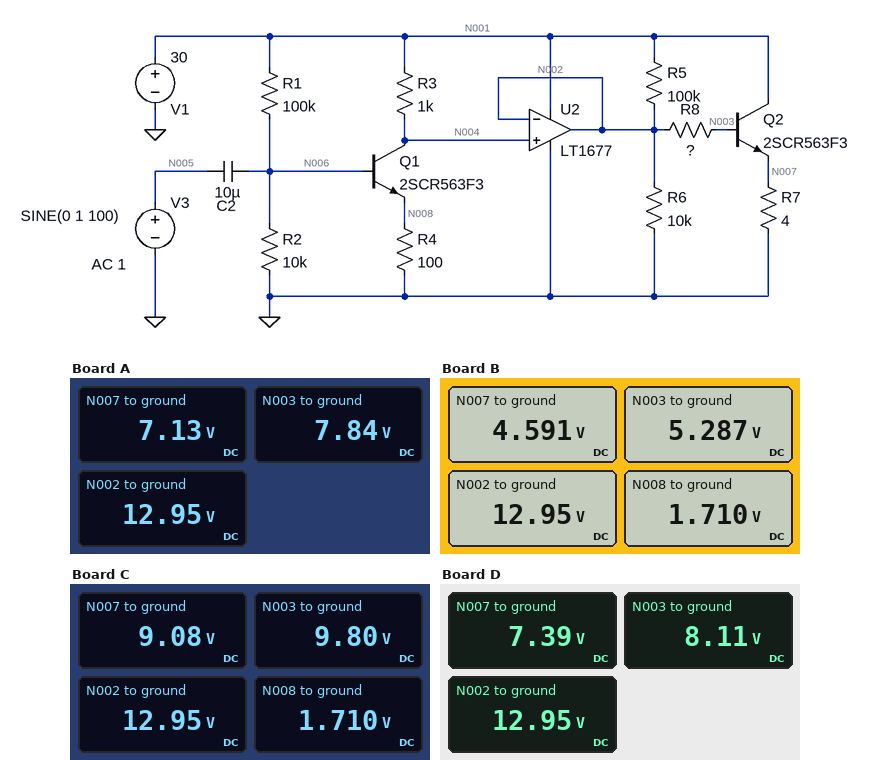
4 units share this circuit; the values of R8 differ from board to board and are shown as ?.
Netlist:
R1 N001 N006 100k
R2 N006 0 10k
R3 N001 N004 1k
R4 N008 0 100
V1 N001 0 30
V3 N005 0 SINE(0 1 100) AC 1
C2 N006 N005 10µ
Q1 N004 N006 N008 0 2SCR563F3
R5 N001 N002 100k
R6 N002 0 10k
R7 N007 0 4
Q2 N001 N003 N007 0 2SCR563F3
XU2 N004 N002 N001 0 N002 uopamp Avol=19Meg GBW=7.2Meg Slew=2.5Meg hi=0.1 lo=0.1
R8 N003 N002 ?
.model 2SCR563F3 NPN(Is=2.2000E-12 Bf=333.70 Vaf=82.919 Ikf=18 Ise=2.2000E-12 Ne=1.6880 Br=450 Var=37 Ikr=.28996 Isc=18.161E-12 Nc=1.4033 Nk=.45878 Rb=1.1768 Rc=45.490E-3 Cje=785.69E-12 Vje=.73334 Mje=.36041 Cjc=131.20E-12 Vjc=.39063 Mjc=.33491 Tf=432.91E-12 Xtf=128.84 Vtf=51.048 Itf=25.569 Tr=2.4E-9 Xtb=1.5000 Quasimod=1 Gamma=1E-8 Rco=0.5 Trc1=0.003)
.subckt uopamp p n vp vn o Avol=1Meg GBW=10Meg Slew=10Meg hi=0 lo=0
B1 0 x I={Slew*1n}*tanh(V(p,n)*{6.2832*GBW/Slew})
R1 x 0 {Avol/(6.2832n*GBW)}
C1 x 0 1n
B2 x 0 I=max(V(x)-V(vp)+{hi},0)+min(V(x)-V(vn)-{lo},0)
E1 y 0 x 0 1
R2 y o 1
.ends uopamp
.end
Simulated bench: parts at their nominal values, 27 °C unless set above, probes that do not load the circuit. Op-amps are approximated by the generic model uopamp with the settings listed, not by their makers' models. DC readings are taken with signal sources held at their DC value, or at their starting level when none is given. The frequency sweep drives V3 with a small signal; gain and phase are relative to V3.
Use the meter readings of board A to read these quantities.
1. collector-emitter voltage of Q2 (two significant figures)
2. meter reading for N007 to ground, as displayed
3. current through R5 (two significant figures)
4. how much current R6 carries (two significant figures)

23 V
7.13 V
170 µA
1.3 mA
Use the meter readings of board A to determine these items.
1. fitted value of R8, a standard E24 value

1.1 kΩ
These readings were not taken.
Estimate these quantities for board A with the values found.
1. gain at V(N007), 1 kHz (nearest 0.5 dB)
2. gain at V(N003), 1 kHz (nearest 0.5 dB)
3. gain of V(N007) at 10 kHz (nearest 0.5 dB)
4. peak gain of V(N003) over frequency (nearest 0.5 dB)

14.5 dB
14.5 dB
14.5 dB
14.5 dB
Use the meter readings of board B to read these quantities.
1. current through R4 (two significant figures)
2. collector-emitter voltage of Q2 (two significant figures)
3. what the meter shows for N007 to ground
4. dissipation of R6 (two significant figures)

17 mA
25 V
4.591 V
17 mW
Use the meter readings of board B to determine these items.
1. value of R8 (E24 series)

2.7 kΩ
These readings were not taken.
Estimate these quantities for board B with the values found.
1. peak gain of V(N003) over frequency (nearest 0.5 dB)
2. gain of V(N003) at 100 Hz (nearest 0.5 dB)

11.0 dB
11.0 dB
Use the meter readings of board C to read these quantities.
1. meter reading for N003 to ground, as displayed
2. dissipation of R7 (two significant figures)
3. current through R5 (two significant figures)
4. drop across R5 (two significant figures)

9.80 V
21 W
170 µA
17 V
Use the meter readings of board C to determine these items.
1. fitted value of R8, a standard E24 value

510 Ω
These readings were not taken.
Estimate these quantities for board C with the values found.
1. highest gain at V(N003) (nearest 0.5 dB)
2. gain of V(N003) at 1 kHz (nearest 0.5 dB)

17.0 dB
17.0 dB
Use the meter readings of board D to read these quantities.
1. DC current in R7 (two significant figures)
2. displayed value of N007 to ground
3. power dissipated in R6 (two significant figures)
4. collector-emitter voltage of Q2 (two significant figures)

1.8 A
7.39 V
17 mW
23 V
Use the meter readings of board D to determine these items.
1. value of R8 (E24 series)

1 kΩ
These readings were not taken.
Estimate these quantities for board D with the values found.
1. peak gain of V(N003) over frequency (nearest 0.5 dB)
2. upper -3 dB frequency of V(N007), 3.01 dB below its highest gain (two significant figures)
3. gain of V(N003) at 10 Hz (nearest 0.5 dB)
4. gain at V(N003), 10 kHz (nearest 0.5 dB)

15.0 dB
940 kHz
14.5 dB
15.0 dB
